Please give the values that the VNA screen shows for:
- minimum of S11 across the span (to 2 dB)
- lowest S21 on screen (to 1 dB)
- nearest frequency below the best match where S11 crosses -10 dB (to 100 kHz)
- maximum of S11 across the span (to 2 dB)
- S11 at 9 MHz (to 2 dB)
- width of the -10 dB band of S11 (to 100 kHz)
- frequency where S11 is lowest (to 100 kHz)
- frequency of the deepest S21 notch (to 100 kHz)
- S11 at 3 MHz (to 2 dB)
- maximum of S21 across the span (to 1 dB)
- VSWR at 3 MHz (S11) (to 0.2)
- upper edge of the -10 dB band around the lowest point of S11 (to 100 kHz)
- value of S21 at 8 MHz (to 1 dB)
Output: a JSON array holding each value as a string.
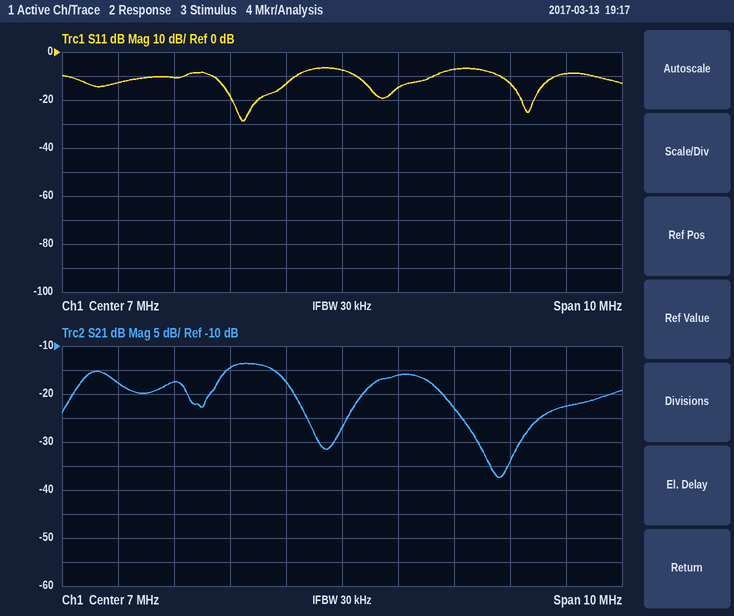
["-28 dB", "-37 dB", "4.7 MHz", "-6 dB", "-8 dB", "1.5 MHz", "5.2 MHz", "9.8 MHz", "-12 dB", "-14 dB", "1.6", "6.2 MHz", "-16 dB"]
